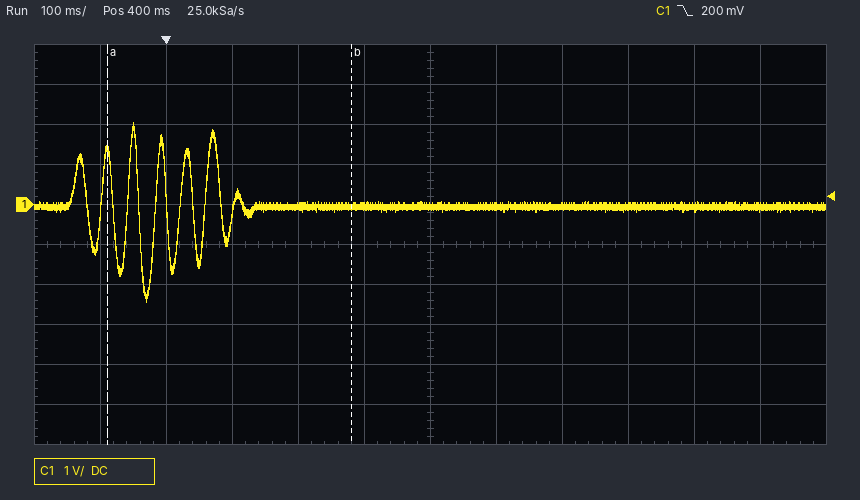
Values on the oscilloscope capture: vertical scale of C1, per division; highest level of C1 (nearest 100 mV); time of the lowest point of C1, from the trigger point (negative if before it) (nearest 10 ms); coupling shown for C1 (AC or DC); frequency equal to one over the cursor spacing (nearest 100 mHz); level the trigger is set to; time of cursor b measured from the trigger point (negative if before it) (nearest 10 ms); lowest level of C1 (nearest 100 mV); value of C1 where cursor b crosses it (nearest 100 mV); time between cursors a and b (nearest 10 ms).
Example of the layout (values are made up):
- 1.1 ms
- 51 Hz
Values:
- 1 V
- 2.0 V
- -30 ms
- DC
- 2.7 Hz
- 200 mV
- +280 ms
- -2.4 V
- -100 mV
- 370 ms
